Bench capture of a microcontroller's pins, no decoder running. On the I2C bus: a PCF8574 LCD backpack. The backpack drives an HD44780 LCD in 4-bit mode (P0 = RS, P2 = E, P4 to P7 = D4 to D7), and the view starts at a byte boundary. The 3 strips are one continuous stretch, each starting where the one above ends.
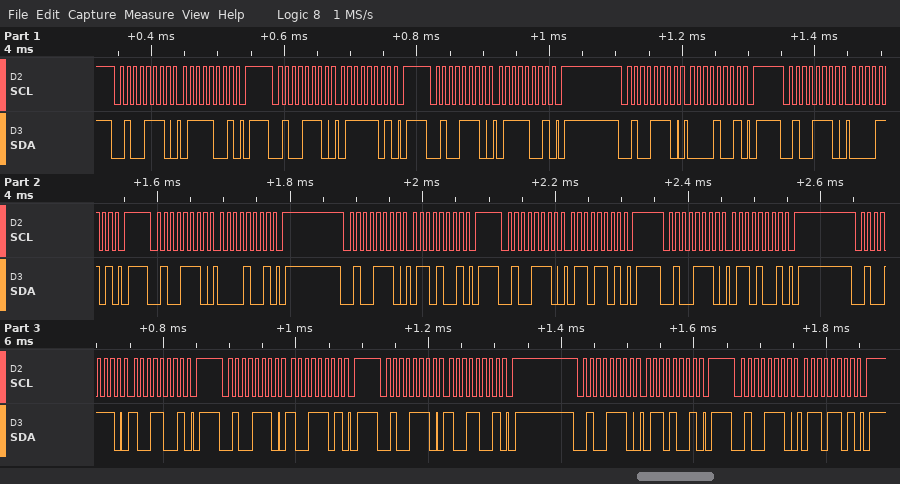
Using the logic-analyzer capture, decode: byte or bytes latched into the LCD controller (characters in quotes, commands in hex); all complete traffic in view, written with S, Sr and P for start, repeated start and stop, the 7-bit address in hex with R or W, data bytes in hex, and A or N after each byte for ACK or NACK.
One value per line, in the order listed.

'p' 'i'
S 27W A 79 A P S 27W A 7D A P S 27W A 79 A P S 27W A 09 A P S 27W A 0D A P S 27W A 09 A P S 27W A 69 A P S 27W A 6D A P S 27W A 69 A P S 27W A 99 A P S 27W A 9D A P S 27W A 99 A P S 27W A 69 A P S 27W A 6D A P
